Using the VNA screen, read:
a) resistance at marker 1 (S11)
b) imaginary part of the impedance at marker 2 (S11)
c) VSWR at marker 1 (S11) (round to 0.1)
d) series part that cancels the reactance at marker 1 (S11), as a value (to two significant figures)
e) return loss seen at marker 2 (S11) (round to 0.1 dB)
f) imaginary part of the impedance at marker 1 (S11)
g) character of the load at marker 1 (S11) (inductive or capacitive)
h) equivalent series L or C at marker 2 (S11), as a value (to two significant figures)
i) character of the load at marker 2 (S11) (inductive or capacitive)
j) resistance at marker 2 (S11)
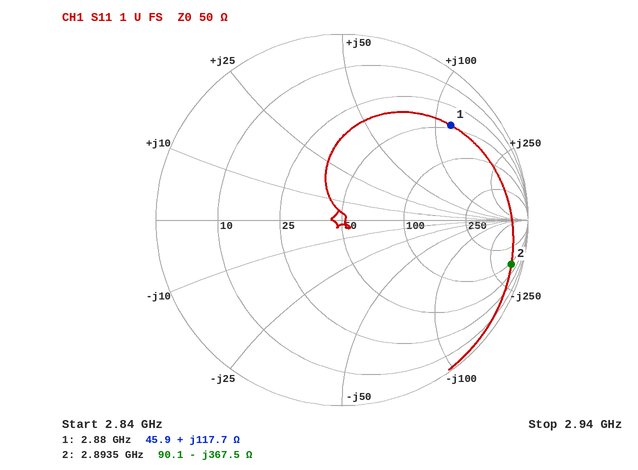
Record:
45.9 Ω
-367.5 Ω
7.9
470 fF
0.5 dB
+117.7 Ω
inductive
150 fF
capacitive
90.1 Ω
